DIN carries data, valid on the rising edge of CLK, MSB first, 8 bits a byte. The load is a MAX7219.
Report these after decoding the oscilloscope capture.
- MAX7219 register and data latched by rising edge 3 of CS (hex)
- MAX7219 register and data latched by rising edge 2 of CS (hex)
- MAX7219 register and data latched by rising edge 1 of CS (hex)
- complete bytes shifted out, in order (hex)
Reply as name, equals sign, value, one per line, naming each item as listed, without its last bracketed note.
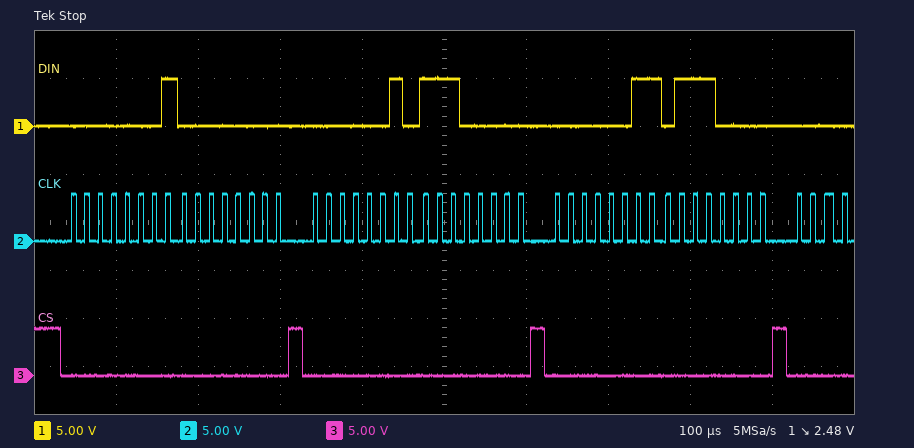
MAX7219 register and data latched by rising edge 3 of CS = register 0x3, data 0x70
MAX7219 register and data latched by rising edge 2 of CS = register 0x2, data 0xE0
MAX7219 register and data latched by rising edge 1 of CS = register 0x1, data 0x00
complete bytes shifted out, in order = 01 00 02 E0 03 70
